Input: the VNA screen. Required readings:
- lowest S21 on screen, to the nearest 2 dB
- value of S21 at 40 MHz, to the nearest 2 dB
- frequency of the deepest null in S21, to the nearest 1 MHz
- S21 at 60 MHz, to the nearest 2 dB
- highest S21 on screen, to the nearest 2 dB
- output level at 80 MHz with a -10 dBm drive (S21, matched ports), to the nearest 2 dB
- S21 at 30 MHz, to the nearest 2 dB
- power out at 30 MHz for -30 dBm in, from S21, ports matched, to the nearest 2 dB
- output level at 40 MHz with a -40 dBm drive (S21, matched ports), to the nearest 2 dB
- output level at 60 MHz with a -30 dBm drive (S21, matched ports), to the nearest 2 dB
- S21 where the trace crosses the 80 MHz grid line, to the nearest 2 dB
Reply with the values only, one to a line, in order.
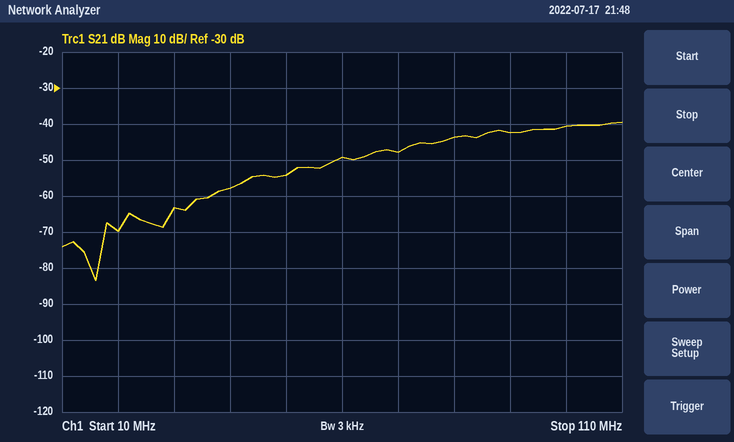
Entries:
-84 dB
-58 dB
16 MHz
-50 dB
-40 dB
-54 dBm
-64 dB
-94 dBm
-98 dBm
-80 dBm
-44 dB
